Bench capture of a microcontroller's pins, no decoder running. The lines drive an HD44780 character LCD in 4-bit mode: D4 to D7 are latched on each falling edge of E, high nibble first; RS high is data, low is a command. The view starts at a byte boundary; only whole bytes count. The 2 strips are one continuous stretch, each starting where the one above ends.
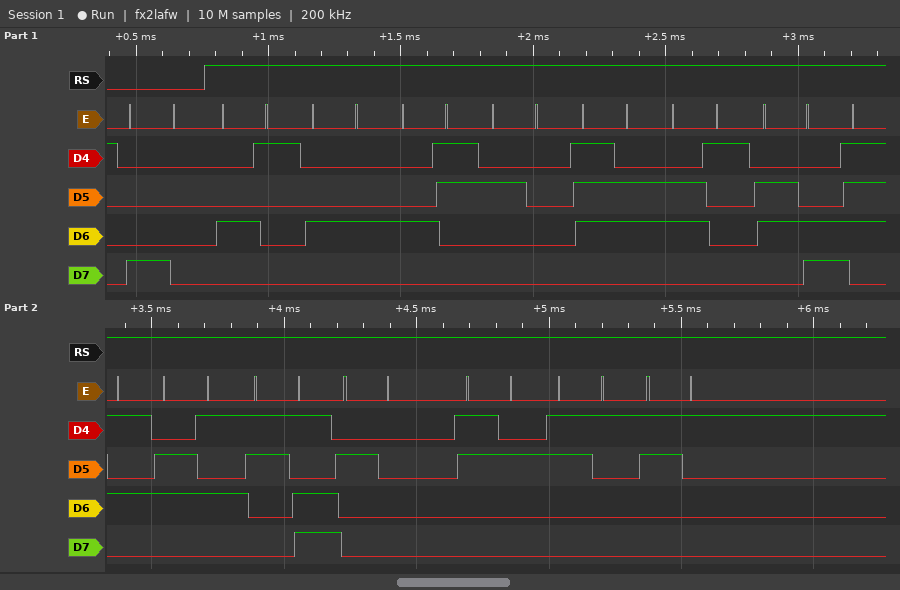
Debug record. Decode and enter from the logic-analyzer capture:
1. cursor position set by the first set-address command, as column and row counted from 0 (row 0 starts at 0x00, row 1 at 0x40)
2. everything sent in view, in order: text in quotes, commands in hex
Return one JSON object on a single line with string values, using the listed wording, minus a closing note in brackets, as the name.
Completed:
{"cursor position set by the first set-address command, as column and row counted from 0": "column 0, row 0", "everything sent in view, in order: text in quotes, commands in hex": "0x80 \"ADC value= 211\""}
